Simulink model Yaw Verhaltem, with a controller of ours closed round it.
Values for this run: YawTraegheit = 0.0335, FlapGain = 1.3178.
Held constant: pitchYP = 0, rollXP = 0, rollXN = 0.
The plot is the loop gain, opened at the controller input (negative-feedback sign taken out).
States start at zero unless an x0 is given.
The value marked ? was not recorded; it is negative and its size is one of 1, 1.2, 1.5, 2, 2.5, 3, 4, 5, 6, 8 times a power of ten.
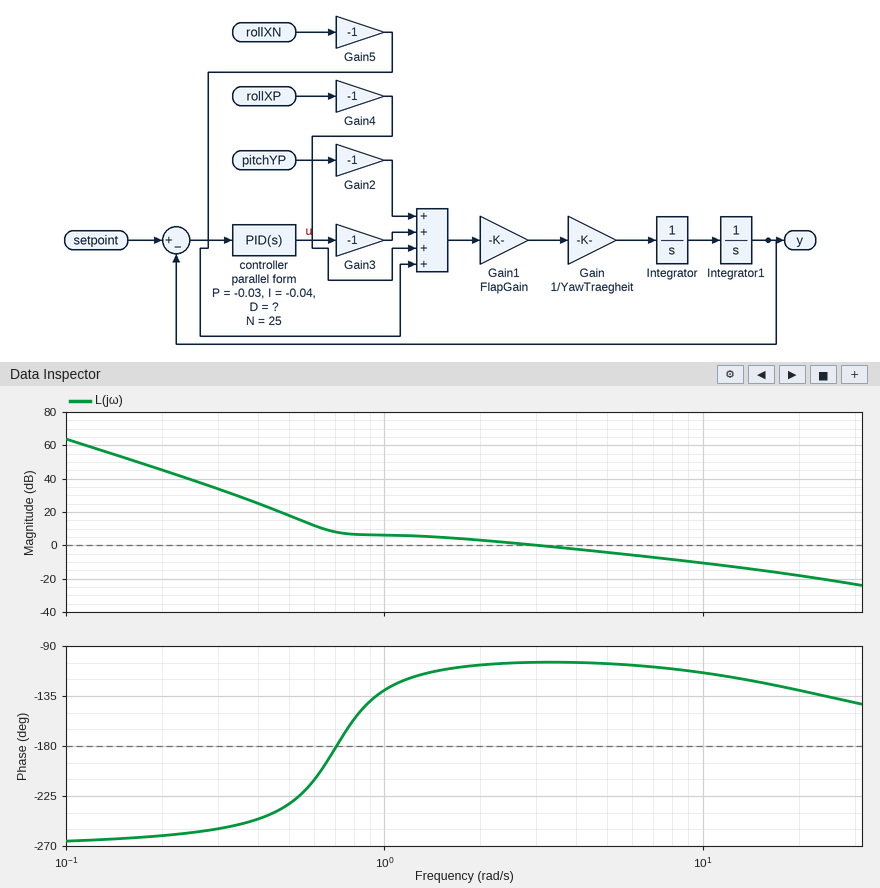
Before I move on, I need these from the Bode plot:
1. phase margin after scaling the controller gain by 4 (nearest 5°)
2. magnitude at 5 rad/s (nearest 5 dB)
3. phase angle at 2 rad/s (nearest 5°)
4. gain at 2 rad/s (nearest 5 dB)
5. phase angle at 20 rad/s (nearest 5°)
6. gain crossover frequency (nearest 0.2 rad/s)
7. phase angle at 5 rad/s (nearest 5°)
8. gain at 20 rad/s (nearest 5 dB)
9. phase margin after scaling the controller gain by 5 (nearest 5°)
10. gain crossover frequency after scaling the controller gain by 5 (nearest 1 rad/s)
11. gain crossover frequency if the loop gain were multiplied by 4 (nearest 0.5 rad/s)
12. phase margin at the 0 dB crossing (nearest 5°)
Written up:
65°
-5 dB
-105°
5 dB
-130°
3.0 rad/s
-105°
-20 dB
60°
14 rad/s
11.5 rad/s
75°
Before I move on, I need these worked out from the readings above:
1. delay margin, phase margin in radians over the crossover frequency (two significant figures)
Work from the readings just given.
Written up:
0.44 s
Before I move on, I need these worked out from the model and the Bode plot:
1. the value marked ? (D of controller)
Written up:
-0.08
